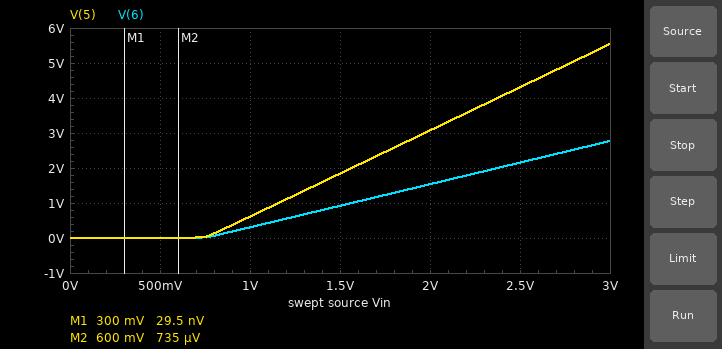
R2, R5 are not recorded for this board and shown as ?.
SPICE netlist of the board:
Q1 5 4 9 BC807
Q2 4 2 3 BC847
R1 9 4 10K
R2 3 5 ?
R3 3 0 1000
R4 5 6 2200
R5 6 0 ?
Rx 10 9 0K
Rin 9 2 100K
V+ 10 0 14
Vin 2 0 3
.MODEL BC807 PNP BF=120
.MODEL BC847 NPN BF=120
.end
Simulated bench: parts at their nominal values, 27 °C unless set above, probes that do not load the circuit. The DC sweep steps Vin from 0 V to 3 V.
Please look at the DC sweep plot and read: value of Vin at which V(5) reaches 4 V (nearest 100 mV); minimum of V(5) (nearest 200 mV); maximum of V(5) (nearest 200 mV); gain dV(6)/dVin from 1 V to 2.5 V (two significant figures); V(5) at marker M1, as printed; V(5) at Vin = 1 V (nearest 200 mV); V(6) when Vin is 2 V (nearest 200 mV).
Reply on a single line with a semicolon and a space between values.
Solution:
2.4 V; 0 V; 5.6 V; 1.2 V/V; 29.5 nV; 600 mV; 1.6 V
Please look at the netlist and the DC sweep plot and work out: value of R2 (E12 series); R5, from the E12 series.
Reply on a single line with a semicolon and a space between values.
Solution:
1.5 kΩ; 2.2 kΩ
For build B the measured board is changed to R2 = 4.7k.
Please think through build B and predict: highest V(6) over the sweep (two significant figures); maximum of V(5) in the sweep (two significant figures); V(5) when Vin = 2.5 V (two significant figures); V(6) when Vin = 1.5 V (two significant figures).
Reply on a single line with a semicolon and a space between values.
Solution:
6.2 V; 12 V; 9.6 V; 2.0 V
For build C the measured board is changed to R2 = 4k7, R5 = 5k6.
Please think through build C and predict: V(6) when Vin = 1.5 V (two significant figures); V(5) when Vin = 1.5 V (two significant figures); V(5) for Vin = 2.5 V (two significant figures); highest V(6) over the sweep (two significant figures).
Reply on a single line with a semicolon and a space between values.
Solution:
2.9 V; 4.1 V; 9.7 V; 9.0 V
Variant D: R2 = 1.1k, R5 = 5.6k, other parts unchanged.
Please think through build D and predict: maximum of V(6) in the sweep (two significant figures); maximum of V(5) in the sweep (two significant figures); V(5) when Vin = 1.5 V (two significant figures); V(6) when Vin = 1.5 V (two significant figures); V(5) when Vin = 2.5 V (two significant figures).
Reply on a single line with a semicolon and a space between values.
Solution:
3.4 V; 4.7 V; 1.6 V; 1.1 V; 3.6 V
